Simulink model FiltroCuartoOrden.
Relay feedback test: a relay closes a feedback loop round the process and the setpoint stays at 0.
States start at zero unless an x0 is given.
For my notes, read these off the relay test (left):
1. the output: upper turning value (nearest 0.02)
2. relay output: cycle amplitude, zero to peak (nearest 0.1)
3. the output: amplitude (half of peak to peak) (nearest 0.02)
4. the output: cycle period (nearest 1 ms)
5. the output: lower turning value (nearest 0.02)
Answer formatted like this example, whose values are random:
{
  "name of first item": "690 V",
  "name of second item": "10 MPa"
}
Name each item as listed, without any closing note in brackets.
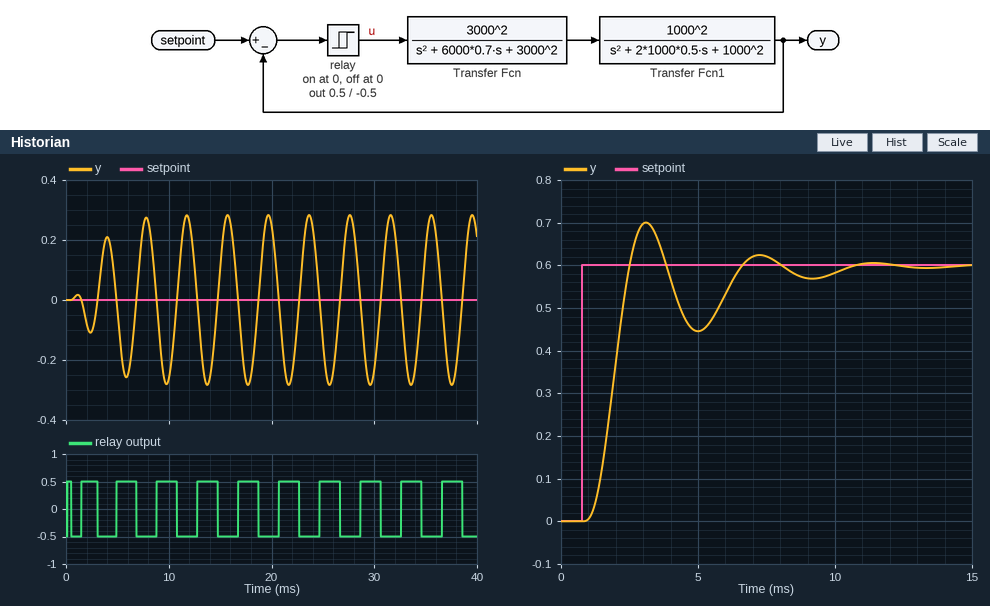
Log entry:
{
  "the output: upper turning value": "0.28",
  "relay output: cycle amplitude, zero to peak": "0.5",
  "the output: amplitude (half of peak to peak)": "0.28",
  "the output: cycle period": "4 ms",
  "the output: lower turning value": "-0.28"
}
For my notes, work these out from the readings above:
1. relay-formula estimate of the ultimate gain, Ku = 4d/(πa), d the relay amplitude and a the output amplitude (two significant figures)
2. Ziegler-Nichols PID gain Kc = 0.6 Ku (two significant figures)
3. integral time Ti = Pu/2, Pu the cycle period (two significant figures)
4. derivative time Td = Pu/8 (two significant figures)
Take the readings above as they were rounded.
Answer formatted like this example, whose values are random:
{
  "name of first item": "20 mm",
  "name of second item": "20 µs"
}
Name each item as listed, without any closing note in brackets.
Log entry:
{
  "relay-formula estimate of the ultimate gain, Ku = 4d/(πa), d the relay amplitude and a the output amplitude": "2.3",
  "Ziegler-Nichols PID gain Kc = 0.6 Ku": "1.4",
  "integral time Ti = Pu/2, Pu the cycle period": "2.0 ms",
  "derivative time Td = Pu/8": "0.50 ms"
}
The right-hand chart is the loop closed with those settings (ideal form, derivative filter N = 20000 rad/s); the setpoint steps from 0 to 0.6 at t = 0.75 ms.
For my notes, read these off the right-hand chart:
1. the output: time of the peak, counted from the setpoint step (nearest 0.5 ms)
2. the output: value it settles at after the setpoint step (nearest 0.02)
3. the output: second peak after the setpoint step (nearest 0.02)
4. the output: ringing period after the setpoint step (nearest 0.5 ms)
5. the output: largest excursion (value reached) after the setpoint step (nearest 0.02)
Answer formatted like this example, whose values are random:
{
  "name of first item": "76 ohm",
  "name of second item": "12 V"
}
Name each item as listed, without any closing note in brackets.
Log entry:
{
  "the output: time of the peak, counted from the setpoint step": "2.5 ms",
  "the output: value it settles at after the setpoint step": "0.60",
  "the output: second peak after the setpoint step": "0.62",
  "the output: ringing period after the setpoint step": "4.0 ms",
  "the output: largest excursion (value reached) after the setpoint step": "0.70"
}
